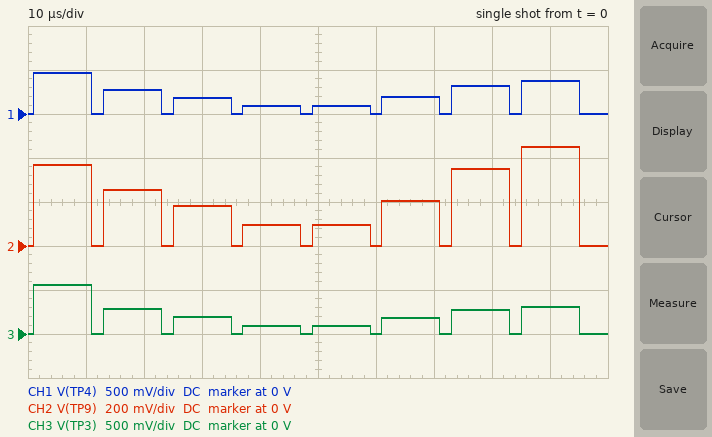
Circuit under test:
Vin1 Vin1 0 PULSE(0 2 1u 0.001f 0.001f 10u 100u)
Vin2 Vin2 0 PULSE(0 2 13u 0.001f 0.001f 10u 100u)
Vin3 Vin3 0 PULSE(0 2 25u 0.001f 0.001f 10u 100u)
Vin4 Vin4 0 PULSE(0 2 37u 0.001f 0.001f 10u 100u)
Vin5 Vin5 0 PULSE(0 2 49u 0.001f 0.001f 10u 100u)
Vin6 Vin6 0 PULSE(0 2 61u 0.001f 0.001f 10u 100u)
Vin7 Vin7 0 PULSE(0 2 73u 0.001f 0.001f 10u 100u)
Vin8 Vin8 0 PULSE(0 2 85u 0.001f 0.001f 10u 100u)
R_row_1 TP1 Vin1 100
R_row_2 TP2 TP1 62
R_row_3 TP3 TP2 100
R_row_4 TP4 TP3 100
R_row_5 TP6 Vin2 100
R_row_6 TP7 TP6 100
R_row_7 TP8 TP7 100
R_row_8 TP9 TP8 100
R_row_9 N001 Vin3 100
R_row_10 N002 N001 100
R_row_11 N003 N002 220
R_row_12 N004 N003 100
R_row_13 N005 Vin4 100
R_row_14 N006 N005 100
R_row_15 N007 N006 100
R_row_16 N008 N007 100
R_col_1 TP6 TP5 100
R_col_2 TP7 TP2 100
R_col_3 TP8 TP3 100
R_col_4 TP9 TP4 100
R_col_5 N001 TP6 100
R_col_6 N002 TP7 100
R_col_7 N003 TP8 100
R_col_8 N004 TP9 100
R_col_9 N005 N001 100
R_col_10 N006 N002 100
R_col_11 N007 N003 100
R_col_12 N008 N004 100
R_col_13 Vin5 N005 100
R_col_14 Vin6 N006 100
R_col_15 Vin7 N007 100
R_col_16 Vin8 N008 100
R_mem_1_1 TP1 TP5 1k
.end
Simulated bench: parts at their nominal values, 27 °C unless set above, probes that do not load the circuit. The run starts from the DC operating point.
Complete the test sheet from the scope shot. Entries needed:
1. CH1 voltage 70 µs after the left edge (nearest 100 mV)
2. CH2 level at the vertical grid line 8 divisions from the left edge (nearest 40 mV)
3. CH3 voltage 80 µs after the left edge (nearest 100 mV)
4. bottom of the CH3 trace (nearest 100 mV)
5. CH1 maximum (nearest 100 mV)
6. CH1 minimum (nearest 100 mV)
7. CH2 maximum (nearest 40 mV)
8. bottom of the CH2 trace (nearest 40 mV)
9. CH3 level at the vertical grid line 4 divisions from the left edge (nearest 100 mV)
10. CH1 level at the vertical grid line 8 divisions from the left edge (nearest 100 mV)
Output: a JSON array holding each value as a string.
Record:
["200 mV", "360 mV", "300 mV", "0 V", "500 mV", "0 V", "440 mV", "0 V", "100 mV", "300 mV"]
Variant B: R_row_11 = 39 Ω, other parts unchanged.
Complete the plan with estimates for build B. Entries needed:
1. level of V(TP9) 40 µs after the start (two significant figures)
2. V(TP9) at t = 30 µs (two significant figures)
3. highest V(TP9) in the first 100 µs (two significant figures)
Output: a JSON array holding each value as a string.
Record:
["110 mV", "210 mV", "410 mV"]
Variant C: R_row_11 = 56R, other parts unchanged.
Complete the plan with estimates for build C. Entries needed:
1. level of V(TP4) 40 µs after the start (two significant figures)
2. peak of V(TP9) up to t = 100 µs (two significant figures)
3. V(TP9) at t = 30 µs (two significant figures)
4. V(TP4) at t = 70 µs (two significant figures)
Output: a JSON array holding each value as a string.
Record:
["100 mV", "420 mV", "200 mV", "210 mV"]
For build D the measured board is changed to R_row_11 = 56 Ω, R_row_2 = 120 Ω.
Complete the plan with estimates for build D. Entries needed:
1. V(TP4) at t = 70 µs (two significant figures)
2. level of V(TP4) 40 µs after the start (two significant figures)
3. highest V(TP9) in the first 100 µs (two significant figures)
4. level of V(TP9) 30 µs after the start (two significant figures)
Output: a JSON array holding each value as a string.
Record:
["220 mV", "110 mV", "430 mV", "210 mV"]
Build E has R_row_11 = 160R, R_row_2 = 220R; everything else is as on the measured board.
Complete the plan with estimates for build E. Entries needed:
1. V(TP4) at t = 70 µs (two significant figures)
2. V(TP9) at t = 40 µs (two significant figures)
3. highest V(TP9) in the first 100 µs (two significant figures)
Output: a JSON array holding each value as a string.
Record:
["220 mV", "110 mV", "470 mV"]
